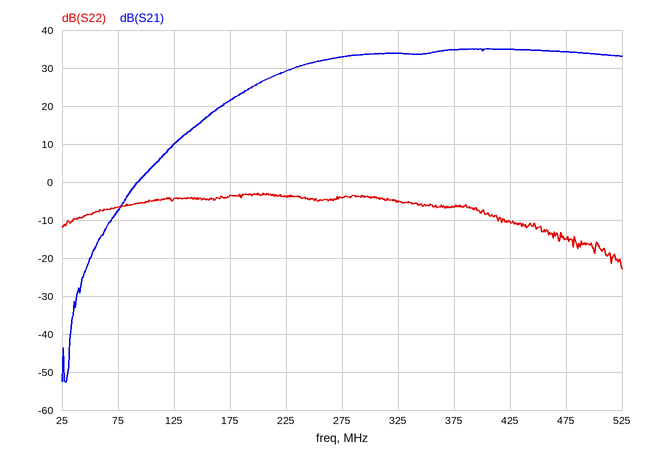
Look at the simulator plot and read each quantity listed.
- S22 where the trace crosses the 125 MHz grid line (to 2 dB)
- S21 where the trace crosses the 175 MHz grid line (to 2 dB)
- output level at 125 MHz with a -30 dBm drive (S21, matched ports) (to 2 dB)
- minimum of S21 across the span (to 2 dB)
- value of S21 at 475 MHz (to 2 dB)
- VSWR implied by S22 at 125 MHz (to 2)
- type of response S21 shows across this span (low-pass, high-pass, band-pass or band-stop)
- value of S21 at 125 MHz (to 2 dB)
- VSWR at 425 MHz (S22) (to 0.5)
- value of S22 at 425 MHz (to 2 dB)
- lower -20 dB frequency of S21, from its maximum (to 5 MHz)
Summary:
-4 dB
22 dB
-20 dBm
-52 dB
34 dB
4
high-pass
10 dB
2.0
-10 dB
145 MHz
